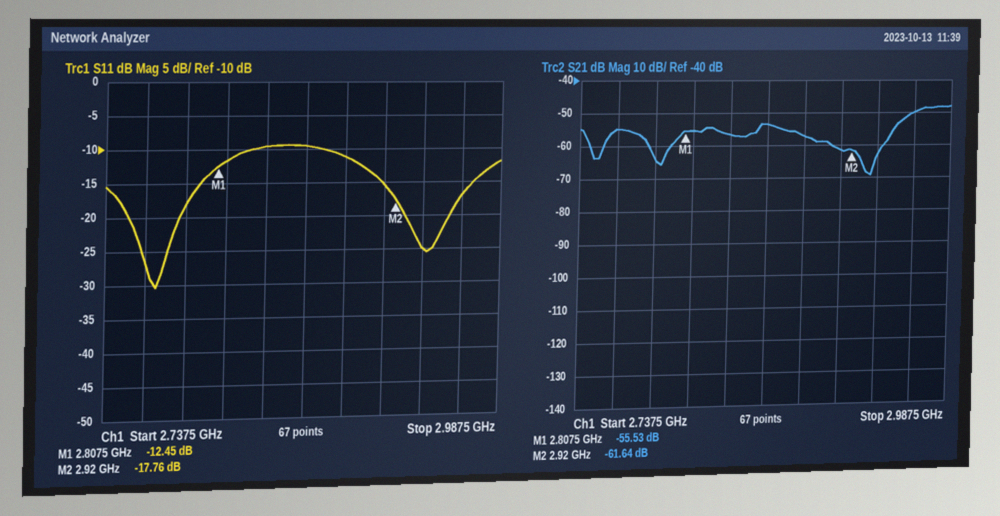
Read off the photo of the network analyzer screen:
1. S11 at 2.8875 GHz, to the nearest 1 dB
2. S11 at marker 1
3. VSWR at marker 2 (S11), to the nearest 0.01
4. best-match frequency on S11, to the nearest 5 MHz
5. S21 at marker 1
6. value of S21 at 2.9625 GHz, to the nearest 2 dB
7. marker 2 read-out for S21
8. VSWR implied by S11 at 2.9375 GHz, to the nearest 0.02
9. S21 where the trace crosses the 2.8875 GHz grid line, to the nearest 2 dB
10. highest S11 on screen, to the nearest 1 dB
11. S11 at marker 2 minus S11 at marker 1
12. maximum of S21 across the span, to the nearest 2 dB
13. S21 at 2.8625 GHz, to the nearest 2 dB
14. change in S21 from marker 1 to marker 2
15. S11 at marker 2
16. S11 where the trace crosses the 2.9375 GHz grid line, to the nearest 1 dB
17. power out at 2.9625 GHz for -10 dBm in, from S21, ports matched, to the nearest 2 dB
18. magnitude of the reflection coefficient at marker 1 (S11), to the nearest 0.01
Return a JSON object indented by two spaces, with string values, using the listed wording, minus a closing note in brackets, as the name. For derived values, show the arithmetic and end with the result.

{
  "S11 at 2.8875 GHz, to the nearest 1 dB": "-11 dB",
  "S11 at marker 1": "-12.45 dB",
  "VSWR at marker 2 (S11), to the nearest 0.01": "(1 + 0.1294)/(1 − 0.1294) ≈ 1.30",
  "best-match frequency on S11, to the nearest 5 MHz": "2.770 GHz",
  "S21 at marker 1": "-55.53 dB",
  "value of S21 at 2.9625 GHz, to the nearest 2 dB": "-50 dB",
  "marker 2 read-out for S21": "-61.64 dB",
  "VSWR implied by S11 at 2.9375 GHz, to the nearest 0.02": "|Γ| = 10^(-25/20) = 0.0562; VSWR = (1 + 0.0562)/(1 − 0.0562) ≈ 1.12",
  "S21 where the trace crosses the 2.8875 GHz grid line, to the nearest 2 dB": "-58 dB",
  "highest S11 on screen, to the nearest 1 dB": "-9 dB",
  "S11 at marker 2 minus S11 at marker 1": "-17.76 − (-12.45) = -5.31 dB",
  "maximum of S21 across the span, to the nearest 2 dB": "-48 dB",
  "S21 at 2.8625 GHz, to the nearest 2 dB": "-54 dB",
  "change in S21 from marker 1 to marker 2": "-61.64 − (-55.53) = -6.11 dB",
  "S11 at marker 2": "-17.76 dB",
  "S11 where the trace crosses the 2.9375 GHz grid line, to the nearest 1 dB": "-25 dB",
  "power out at 2.9625 GHz for -10 dBm in, from S21, ports matched, to the nearest 2 dB": "-10 dBm + (-50 dB) = -60 dBm",
  "magnitude of the reflection coefficient at marker 1 (S11), to the nearest 0.01": "10^(-12.45/20) ≈ 0.24"
}
